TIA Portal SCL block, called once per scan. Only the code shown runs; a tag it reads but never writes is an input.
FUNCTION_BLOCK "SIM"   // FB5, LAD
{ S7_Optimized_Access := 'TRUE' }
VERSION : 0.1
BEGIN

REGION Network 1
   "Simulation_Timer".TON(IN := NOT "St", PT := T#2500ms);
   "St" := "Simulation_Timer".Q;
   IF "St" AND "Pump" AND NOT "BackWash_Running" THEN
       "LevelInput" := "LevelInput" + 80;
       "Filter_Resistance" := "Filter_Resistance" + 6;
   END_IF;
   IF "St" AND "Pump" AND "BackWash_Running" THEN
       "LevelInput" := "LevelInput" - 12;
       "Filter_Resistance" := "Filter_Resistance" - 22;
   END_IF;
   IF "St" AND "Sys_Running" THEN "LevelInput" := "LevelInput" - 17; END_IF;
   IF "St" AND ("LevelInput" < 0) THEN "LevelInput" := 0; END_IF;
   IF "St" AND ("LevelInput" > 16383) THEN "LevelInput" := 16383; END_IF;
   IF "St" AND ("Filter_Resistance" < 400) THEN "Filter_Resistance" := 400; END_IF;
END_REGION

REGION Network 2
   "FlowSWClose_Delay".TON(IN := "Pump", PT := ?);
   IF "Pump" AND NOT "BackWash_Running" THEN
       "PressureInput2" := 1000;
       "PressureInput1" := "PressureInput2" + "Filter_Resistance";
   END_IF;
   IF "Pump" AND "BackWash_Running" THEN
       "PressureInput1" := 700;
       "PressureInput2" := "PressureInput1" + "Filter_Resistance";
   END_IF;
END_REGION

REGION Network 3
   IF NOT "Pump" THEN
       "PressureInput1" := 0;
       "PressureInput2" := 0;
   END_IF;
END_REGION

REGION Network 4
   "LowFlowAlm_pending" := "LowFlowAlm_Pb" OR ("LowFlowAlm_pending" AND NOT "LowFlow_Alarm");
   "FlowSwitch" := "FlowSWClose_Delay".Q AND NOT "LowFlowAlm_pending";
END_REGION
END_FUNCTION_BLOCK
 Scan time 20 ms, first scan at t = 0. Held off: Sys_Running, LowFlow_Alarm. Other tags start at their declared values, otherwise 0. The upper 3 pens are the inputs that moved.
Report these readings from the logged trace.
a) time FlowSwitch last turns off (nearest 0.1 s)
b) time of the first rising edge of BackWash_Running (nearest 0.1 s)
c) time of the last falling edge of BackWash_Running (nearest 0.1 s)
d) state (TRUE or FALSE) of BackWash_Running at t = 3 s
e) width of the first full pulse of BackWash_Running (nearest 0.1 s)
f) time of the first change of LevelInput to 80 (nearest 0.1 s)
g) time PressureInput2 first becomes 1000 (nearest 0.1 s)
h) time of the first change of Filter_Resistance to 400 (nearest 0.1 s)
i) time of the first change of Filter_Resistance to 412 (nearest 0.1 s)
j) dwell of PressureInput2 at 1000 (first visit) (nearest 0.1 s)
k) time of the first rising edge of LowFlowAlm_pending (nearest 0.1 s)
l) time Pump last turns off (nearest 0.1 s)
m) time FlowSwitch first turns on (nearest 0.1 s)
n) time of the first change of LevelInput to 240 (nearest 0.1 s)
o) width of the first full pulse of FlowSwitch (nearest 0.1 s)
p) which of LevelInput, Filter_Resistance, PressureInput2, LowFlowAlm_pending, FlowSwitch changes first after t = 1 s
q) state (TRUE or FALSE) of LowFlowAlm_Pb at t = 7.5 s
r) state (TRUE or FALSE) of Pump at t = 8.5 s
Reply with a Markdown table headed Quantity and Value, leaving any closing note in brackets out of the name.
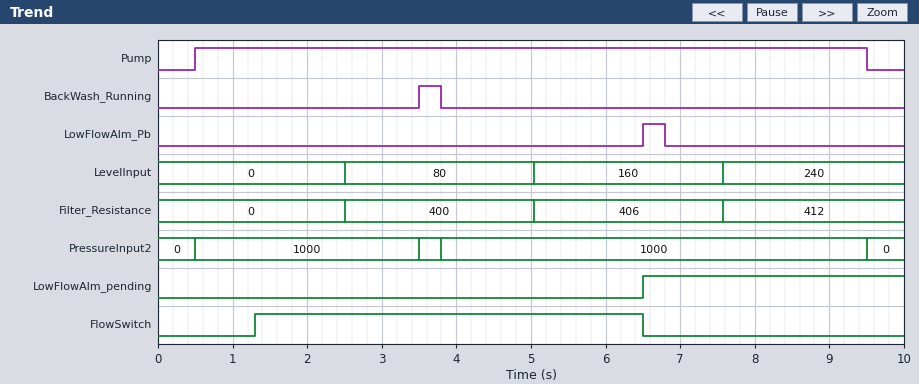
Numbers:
| Quantity | Value |
|---|---|
| time FlowSwitch last turns off | 6.5 s |
| time of the first rising edge of BackWash_Running | 3.5 s |
| time of the last falling edge of BackWash_Running | 3.8 s |
| state (TRUE or FALSE) of BackWash_Running at t = 3 s | FALSE |
| width of the first full pulse of BackWash_Running | 0.3 s |
| time of the first change of LevelInput to 80 | 2.5 s |
| time PressureInput2 first becomes 1000 | 0.5 s |
| time of the first change of Filter_Resistance to 400 | 2.5 s |
| time of the first change of Filter_Resistance to 412 | 7.6 s |
| dwell of PressureInput2 at 1000 (first visit) | 3.0 s |
| time of the first rising edge of LowFlowAlm_pending | 6.5 s |
| time Pump last turns off | 9.5 s |
| time FlowSwitch first turns on | 1.3 s |
| time of the first change of LevelInput to 240 | 7.6 s |
| width of the first full pulse of FlowSwitch | 5.2 s |
| which of LevelInput, Filter_Resistance, PressureInput2, LowFlowAlm_pending, FlowSwitch changes first after t = 1 s | FlowSwitch |
| state (TRUE or FALSE) of LowFlowAlm_Pb at t = 7.5 s | FALSE |
| state (TRUE or FALSE) of Pump at t = 8.5 s | TRUE |
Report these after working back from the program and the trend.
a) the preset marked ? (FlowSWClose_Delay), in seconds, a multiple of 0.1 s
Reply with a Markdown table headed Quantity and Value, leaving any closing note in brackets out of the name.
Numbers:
| Quantity | Value |
|---|---|
| the preset marked ? (FlowSWClose_Delay), in seconds, a multiple of 0.1 s | 0.8 s |
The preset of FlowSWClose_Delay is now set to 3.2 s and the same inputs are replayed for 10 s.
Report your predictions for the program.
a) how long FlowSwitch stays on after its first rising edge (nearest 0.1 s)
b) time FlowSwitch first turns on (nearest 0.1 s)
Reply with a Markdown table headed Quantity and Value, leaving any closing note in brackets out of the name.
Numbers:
| Quantity | Value |
|---|---|
| how long FlowSwitch stays on after its first rising edge | 2.8 s |
| time FlowSwitch first turns on | 3.7 s |
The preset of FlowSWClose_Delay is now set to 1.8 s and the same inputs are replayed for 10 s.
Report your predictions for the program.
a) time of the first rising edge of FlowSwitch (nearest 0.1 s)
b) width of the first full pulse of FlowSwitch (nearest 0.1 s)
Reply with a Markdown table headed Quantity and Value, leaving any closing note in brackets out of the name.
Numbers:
| Quantity | Value |
|---|---|
| time of the first rising edge of FlowSwitch | 2.3 s |
| width of the first full pulse of FlowSwitch | 4.2 s |
